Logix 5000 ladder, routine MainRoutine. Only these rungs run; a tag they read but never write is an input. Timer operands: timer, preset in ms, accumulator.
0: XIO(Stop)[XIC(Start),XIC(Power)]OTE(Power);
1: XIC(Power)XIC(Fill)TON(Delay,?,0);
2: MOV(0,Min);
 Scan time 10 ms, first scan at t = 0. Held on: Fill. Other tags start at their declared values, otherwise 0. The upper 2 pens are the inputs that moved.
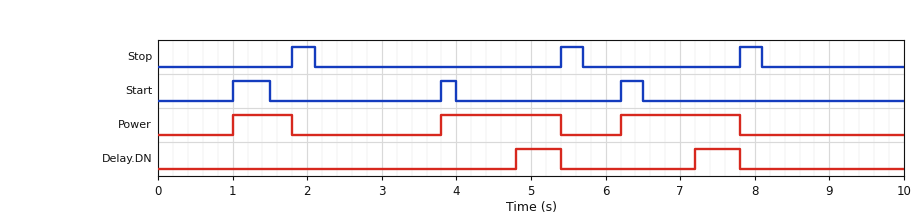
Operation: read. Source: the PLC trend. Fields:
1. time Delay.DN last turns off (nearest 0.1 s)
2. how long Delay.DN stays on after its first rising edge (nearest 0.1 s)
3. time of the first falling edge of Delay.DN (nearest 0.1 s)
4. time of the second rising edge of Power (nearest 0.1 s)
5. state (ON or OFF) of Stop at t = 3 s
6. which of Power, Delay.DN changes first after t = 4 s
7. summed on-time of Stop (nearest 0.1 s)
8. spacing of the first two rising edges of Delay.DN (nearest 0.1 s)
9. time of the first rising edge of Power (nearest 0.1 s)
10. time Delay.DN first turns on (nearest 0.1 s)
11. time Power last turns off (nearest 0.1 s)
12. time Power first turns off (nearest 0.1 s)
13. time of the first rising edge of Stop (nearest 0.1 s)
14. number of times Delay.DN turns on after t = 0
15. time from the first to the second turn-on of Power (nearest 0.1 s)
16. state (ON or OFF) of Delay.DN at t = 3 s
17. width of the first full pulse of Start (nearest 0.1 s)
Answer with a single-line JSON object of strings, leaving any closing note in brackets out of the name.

{"time Delay.DN last turns off": "7.8 s", "how long Delay.DN stays on after its first rising edge": "0.6 s", "time of the first falling edge of Delay.DN": "5.4 s", "time of the second rising edge of Power": "3.8 s", "state (ON or OFF) of Stop at t = 3 s": "OFF", "which of Power, Delay.DN changes first after t = 4 s": "Delay.DN", "summed on-time of Stop": "0.9 s", "spacing of the first two rising edges of Delay.DN": "2.4 s", "time of the first rising edge of Power": "1.0 s", "time Delay.DN first turns on": "4.8 s", "time Power last turns off": "7.8 s", "time Power first turns off": "1.8 s", "time of the first rising edge of Stop": "1.8 s", "number of times Delay.DN turns on after t = 0": "2", "time from the first to the second turn-on of Power": "2.8 s", "state (ON or OFF) of Delay.DN at t = 3 s": "OFF", "width of the first full pulse of Start": "0.5 s"}
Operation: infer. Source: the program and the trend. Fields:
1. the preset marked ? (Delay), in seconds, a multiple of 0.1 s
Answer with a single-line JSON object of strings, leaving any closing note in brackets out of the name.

{"the preset marked ? (Delay), in seconds, a multiple of 0.1 s": "1.0 s"}
